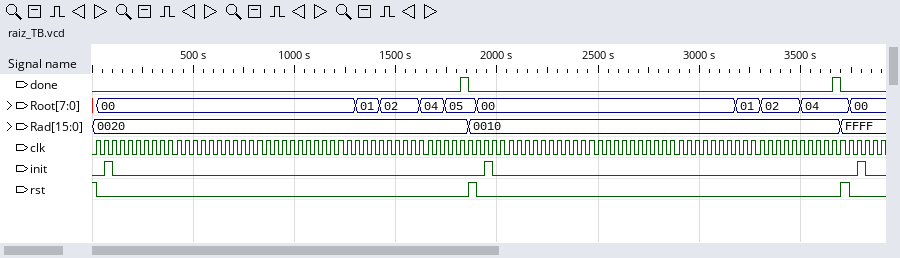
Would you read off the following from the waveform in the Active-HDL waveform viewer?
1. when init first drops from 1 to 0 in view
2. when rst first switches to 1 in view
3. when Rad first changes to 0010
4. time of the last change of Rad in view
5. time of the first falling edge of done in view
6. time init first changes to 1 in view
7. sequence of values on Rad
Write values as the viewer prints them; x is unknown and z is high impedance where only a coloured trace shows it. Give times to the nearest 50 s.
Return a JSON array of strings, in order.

["100 s", "1850 s", "1850 s", "3700 s", "1850 s", "50 s", "0020, 0010, FFFF"]
